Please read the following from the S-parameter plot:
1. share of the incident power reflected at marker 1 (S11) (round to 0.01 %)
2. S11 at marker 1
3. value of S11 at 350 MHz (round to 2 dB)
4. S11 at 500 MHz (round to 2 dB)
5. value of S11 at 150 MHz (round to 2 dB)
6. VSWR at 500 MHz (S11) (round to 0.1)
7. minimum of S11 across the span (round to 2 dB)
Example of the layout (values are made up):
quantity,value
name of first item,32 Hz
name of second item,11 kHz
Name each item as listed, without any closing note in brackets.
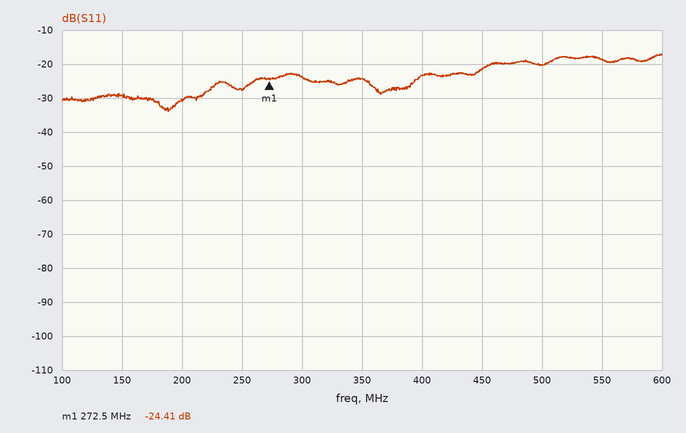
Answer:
quantity,value
share of the incident power reflected at marker 1 (S11),0.36 %
S11 at marker 1,-24.41 dB
value of S11 at 350 MHz,-24 dB
S11 at 500 MHz,-20 dB
value of S11 at 150 MHz,-30 dB
VSWR at 500 MHz (S11),1.2
minimum of S11 across the span,-34 dB
